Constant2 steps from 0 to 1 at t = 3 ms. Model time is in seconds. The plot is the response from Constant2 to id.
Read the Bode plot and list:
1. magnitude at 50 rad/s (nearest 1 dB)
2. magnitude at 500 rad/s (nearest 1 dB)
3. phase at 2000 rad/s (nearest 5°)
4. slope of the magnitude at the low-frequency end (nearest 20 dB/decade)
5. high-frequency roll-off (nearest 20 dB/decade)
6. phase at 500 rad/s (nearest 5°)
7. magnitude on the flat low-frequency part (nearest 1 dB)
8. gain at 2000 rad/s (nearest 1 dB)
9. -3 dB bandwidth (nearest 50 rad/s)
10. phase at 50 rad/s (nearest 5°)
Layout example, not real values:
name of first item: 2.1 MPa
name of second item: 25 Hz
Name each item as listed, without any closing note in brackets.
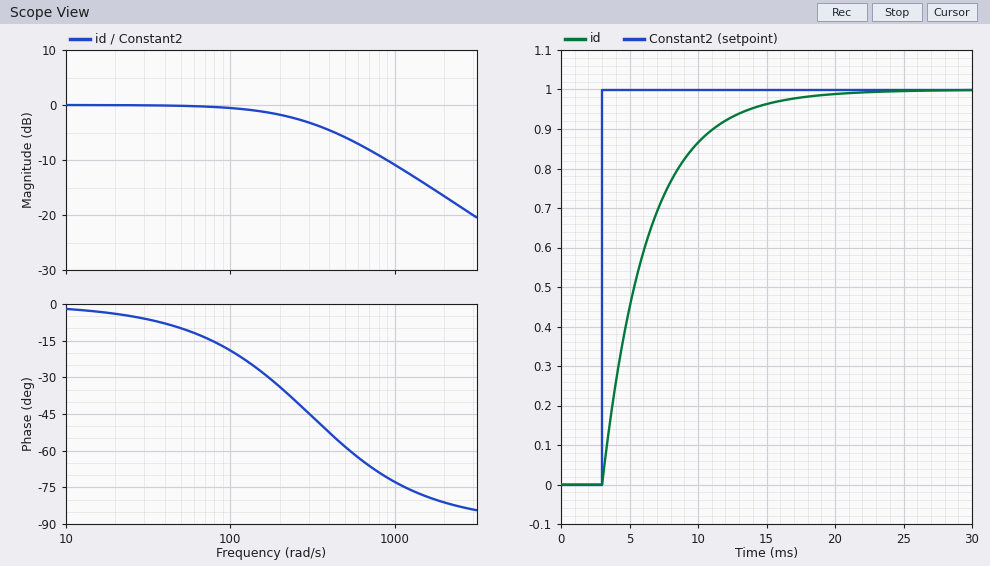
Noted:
magnitude at 50 rad/s: 0 dB
magnitude at 500 rad/s: -6 dB
phase at 2000 rad/s: -80°
slope of the magnitude at the low-frequency end: 0 dB/decade
high-frequency roll-off: -20 dB/decade
phase at 500 rad/s: -60°
magnitude on the flat low-frequency part: 0 dB
gain at 2000 rad/s: -17 dB
-3 dB bandwidth: 300 rad/s
phase at 50 rad/s: -10°
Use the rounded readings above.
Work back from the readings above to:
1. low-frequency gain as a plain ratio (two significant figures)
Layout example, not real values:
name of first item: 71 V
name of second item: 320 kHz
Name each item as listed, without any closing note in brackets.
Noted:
low-frequency gain as a plain ratio: 1.0
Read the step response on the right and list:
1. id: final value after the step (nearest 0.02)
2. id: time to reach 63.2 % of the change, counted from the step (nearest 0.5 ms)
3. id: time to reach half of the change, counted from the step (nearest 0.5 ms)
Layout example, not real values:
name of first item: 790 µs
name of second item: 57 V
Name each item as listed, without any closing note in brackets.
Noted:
id: final value after the step: 1.00
id: time to reach 63.2 % of the change, counted from the step: 3.5 ms
id: time to reach half of the change, counted from the step: 2.5 ms
